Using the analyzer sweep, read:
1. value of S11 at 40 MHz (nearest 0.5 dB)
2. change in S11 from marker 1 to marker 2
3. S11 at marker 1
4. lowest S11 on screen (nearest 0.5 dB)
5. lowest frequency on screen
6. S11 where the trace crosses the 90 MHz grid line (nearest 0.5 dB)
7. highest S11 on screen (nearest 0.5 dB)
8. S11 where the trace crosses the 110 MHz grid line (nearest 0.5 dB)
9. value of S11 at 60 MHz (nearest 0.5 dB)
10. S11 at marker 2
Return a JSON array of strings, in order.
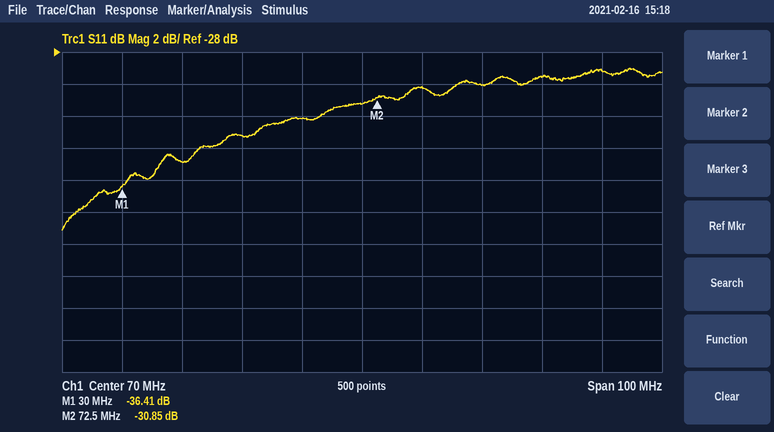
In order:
["-35.0 dB", "5.56 dB", "-36.41 dB", "-39.0 dB", "20 MHz", "-30.0 dB", "-29.0 dB", "-29.0 dB", "-32.0 dB", "-30.85 dB"]
